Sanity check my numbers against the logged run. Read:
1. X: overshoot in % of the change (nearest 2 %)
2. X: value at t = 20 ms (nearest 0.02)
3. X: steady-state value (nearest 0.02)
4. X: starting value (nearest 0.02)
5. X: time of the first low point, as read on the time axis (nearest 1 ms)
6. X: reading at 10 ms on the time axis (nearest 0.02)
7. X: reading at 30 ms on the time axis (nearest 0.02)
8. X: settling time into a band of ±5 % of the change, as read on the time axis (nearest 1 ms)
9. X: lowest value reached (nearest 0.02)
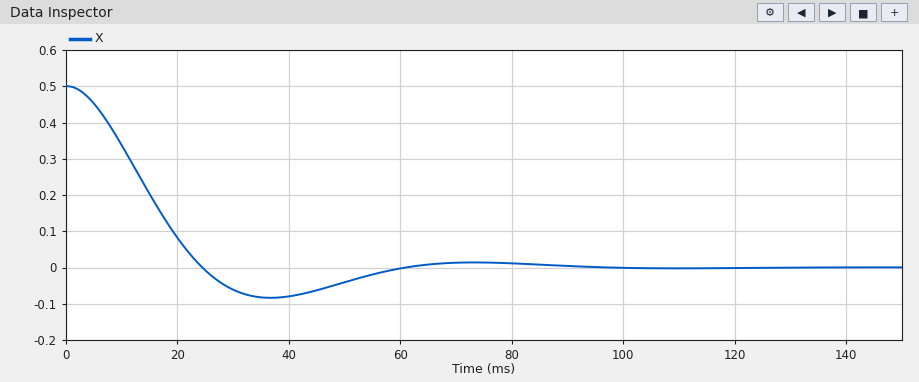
16 %
0.08
0.00
0.50
37 ms
0.34
-0.06
54 ms
-0.08
